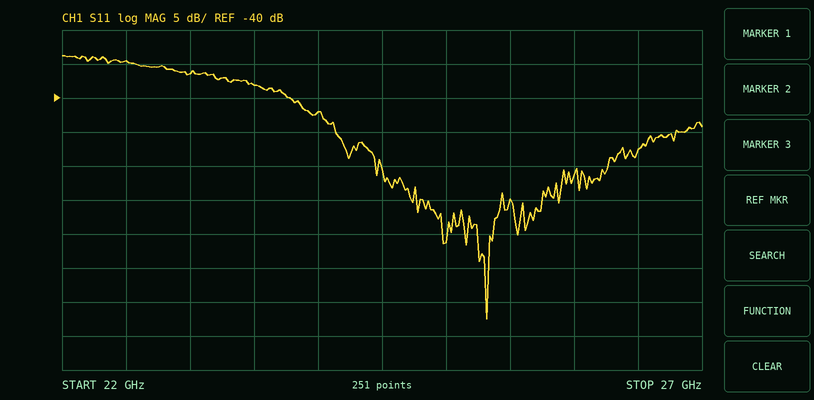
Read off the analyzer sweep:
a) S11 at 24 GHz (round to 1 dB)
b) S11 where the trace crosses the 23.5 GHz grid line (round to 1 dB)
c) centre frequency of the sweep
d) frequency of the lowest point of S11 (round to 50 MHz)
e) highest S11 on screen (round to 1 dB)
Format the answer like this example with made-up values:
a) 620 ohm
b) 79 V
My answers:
a) -42 dB
b) -38 dB
c) 24.5 GHz
d) 25.30 GHz
e) -34 dB
